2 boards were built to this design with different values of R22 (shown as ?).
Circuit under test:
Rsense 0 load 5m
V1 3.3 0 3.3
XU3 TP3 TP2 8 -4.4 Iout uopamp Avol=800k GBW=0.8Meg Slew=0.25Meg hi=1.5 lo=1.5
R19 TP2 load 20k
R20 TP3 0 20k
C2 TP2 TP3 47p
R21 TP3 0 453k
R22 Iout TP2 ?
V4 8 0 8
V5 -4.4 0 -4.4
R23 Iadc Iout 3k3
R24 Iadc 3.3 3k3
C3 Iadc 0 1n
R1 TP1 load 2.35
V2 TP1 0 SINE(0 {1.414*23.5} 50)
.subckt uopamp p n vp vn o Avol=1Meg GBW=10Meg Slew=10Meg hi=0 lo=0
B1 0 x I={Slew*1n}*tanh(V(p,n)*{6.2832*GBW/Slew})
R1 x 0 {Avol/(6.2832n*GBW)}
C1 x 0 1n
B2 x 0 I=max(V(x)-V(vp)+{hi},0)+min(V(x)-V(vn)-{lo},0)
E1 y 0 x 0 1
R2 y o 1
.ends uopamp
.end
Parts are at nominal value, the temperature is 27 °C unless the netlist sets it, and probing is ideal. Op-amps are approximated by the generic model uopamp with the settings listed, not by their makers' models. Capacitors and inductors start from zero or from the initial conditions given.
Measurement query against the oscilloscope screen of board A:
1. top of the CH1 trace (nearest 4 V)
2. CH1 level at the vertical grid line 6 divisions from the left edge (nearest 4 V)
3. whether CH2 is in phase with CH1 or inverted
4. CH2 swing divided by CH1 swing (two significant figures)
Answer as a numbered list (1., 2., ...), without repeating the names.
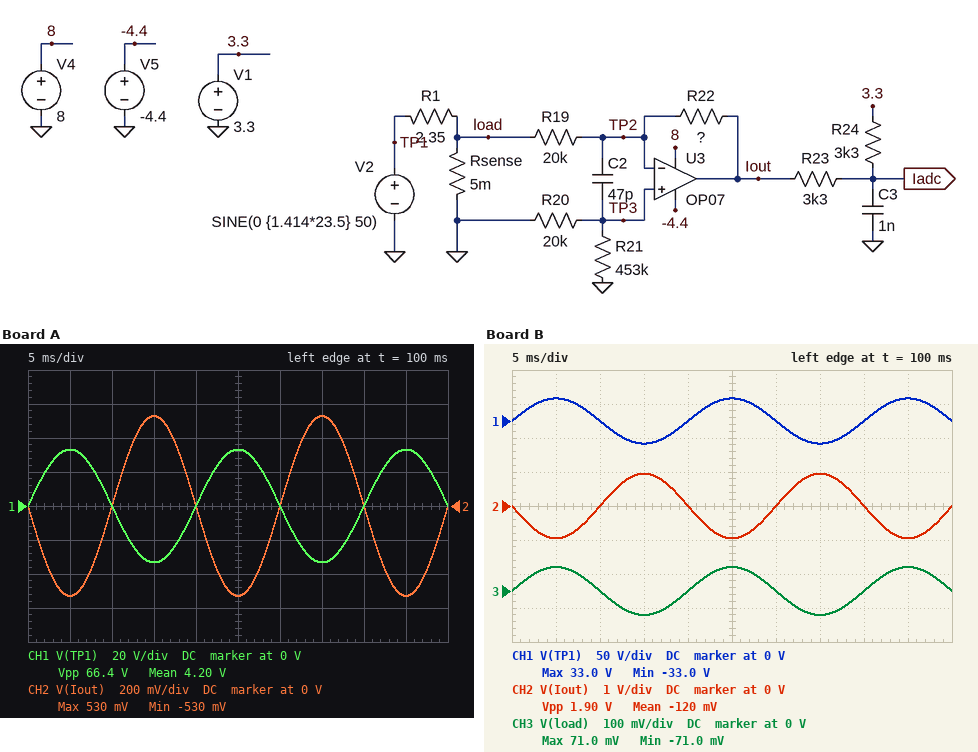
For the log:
1. 32 V
2. 0 V
3. inverted
4. 0.016
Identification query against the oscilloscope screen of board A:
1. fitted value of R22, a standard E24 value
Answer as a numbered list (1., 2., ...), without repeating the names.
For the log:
1. 150 kΩ
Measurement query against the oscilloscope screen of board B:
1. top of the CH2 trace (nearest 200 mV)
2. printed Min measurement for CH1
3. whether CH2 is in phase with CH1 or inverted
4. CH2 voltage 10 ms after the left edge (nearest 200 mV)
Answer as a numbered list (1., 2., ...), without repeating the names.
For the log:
1. 1.0 V
2. -33.0 V
3. inverted
4. 0 V
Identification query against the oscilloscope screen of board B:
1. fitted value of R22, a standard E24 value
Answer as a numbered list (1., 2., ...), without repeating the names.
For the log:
1. 270 kΩ
